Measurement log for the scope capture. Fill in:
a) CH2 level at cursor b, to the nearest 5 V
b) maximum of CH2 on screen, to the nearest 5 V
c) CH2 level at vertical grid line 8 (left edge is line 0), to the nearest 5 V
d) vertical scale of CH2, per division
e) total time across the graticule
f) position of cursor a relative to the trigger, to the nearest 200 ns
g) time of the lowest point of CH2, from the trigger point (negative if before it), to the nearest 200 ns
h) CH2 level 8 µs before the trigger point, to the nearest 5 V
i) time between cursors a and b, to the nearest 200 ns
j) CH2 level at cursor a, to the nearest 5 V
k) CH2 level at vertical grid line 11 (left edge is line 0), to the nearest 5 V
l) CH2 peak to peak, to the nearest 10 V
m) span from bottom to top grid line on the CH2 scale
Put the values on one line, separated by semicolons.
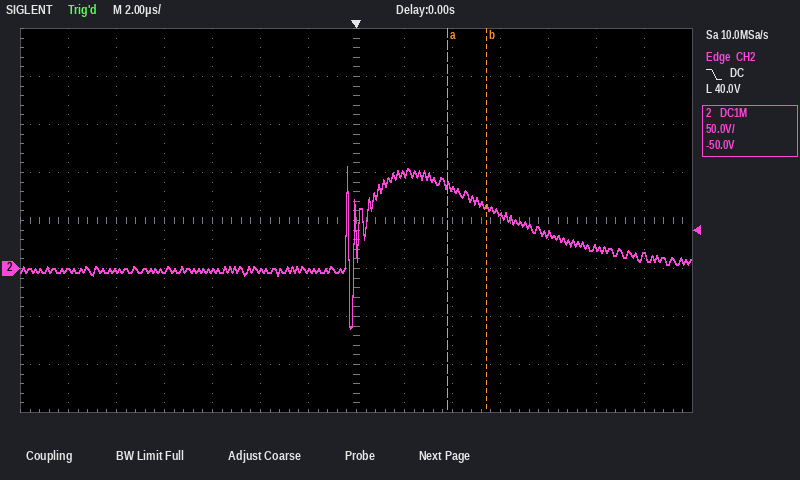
65 V; 105 V; 100 V; 50 V; 28 µs; +3.8 µs; -200 ns; -5 V; 1.6 µs; 85 V; 35 V; 170 V; 400 V
